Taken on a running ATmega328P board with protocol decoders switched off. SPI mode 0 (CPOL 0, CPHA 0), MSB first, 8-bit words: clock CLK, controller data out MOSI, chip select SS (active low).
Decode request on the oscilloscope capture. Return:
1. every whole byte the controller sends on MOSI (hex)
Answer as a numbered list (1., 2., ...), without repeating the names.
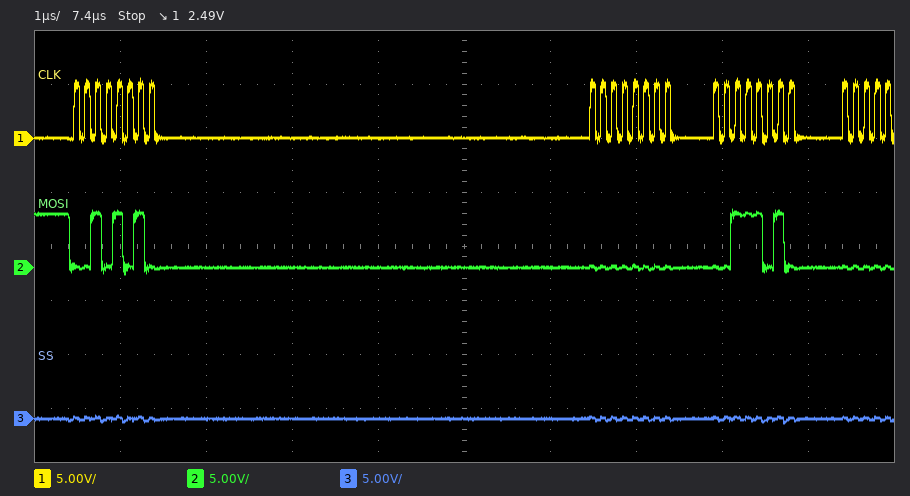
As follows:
1. 2A 00 3A
